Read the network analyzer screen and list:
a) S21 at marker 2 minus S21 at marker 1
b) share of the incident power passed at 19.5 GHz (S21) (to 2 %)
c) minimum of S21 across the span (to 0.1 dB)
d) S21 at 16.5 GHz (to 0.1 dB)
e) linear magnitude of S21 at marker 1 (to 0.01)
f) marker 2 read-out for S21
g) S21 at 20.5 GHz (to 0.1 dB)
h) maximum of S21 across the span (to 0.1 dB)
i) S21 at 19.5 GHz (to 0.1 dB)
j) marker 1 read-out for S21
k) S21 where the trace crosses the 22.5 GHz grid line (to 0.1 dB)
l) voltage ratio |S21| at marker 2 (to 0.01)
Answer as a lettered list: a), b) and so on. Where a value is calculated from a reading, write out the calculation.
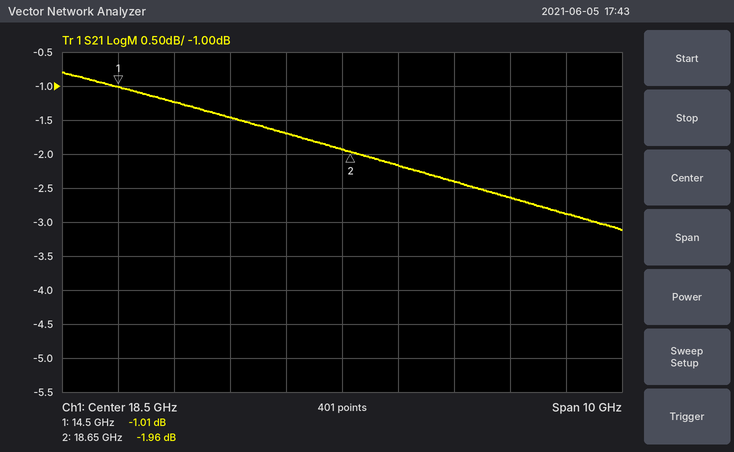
a) -1.96 − (-1.01) = -0.95 dB
b) 10^(-2.2/10) ≈ 60 %
c) -3.1 dB
d) -1.5 dB
e) 10^(-1.01/20) ≈ 0.89
f) -1.96 dB
g) -2.4 dB
h) -0.8 dB
i) -2.2 dB
j) -1.01 dB
k) -2.9 dB
l) 10^(-1.96/20) ≈ 0.80
